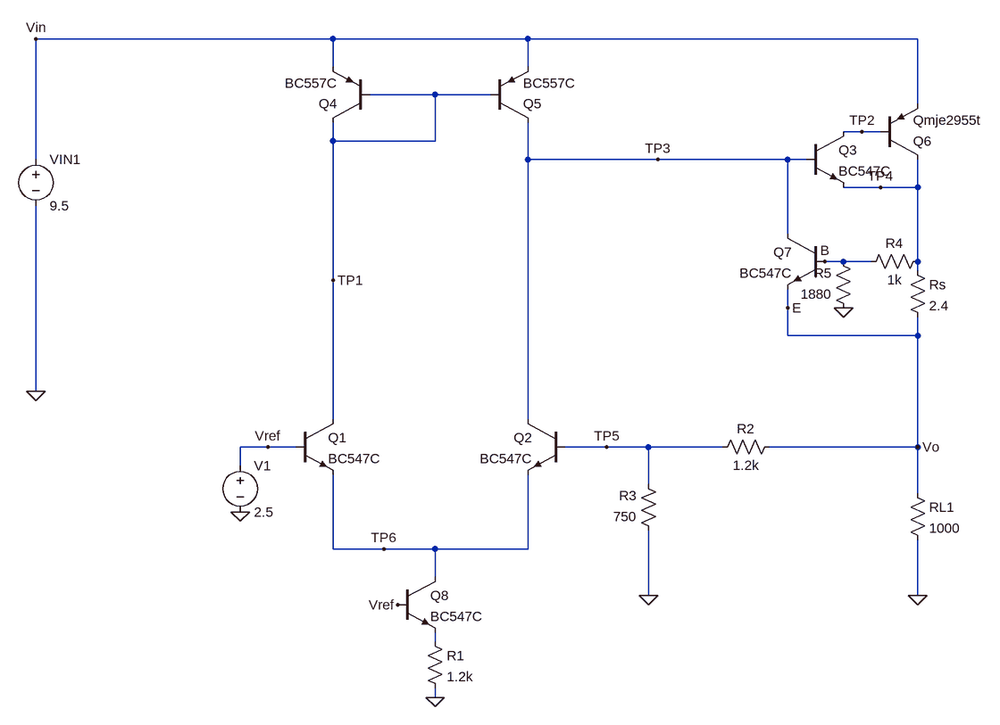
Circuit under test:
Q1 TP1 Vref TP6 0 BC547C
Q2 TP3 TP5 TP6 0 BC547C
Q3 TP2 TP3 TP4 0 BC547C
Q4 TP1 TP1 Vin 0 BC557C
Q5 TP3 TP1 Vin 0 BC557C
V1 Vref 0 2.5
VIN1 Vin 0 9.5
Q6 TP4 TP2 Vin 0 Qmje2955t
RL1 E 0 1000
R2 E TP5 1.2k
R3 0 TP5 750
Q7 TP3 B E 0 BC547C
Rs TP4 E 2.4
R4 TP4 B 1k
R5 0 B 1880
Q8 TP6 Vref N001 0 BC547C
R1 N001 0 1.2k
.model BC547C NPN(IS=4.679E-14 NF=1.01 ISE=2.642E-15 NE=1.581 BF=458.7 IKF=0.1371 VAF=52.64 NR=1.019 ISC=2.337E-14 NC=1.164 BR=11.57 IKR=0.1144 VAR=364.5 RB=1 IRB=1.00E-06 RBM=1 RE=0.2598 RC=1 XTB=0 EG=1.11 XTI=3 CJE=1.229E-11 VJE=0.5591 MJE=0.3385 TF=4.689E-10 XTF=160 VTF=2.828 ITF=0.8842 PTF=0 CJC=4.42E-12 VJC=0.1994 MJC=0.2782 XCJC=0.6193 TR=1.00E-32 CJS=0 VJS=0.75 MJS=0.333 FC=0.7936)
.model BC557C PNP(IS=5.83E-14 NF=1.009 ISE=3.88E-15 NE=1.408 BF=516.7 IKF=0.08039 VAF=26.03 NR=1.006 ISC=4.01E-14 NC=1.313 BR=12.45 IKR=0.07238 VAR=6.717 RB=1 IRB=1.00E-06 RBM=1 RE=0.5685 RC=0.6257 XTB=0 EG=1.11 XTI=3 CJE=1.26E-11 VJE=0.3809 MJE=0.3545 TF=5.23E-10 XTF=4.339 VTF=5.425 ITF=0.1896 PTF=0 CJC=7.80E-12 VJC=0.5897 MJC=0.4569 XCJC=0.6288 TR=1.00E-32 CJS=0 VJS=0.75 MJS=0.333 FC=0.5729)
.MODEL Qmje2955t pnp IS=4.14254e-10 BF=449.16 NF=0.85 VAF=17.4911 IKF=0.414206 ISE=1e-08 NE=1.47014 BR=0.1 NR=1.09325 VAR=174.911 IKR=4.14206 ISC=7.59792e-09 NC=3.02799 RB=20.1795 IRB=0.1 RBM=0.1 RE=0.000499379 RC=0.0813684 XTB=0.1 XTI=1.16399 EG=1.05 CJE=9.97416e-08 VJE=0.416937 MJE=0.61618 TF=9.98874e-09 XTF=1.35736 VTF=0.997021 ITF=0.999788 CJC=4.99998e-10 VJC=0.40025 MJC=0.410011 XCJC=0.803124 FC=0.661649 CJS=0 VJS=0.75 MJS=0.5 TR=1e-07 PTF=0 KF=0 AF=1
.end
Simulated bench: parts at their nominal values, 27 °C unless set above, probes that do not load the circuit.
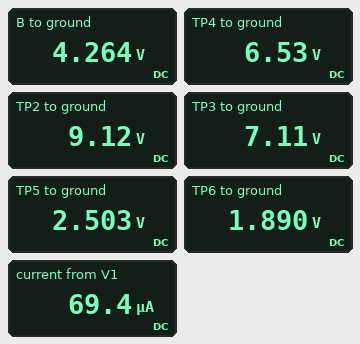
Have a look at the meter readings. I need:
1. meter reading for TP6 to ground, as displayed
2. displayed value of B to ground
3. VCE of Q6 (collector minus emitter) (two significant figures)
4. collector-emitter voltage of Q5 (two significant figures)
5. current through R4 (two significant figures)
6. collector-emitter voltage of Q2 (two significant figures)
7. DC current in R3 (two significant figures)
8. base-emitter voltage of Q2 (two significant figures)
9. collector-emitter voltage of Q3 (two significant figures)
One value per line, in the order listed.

1.890 V
4.264 V
-3.0 V
-2.4 V
2.3 mA
5.2 V
3.3 mA
610 mV
2.6 V
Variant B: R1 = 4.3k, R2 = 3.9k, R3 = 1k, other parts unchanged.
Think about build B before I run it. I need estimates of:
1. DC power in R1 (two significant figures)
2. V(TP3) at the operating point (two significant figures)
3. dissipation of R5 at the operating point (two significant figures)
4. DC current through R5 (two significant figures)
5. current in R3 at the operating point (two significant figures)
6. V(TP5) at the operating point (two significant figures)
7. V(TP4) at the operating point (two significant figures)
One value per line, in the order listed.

830 µW
9.5 V
18 mW
3.1 mA
1.8 mA
1.8 V
8.9 V
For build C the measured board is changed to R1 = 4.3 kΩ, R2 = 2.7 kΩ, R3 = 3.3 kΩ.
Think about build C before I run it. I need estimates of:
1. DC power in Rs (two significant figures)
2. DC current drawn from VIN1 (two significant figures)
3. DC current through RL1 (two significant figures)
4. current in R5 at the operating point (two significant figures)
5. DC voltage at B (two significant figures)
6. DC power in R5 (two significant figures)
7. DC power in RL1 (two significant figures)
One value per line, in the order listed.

68 µW
7.3 mA
4.6 mA
1.6 mA
3.0 V
4.7 mW
21 mW
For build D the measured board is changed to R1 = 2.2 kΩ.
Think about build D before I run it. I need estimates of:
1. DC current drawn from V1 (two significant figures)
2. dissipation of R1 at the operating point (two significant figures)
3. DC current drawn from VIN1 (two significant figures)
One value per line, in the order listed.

38 µA
1.6 mW
13 mA
